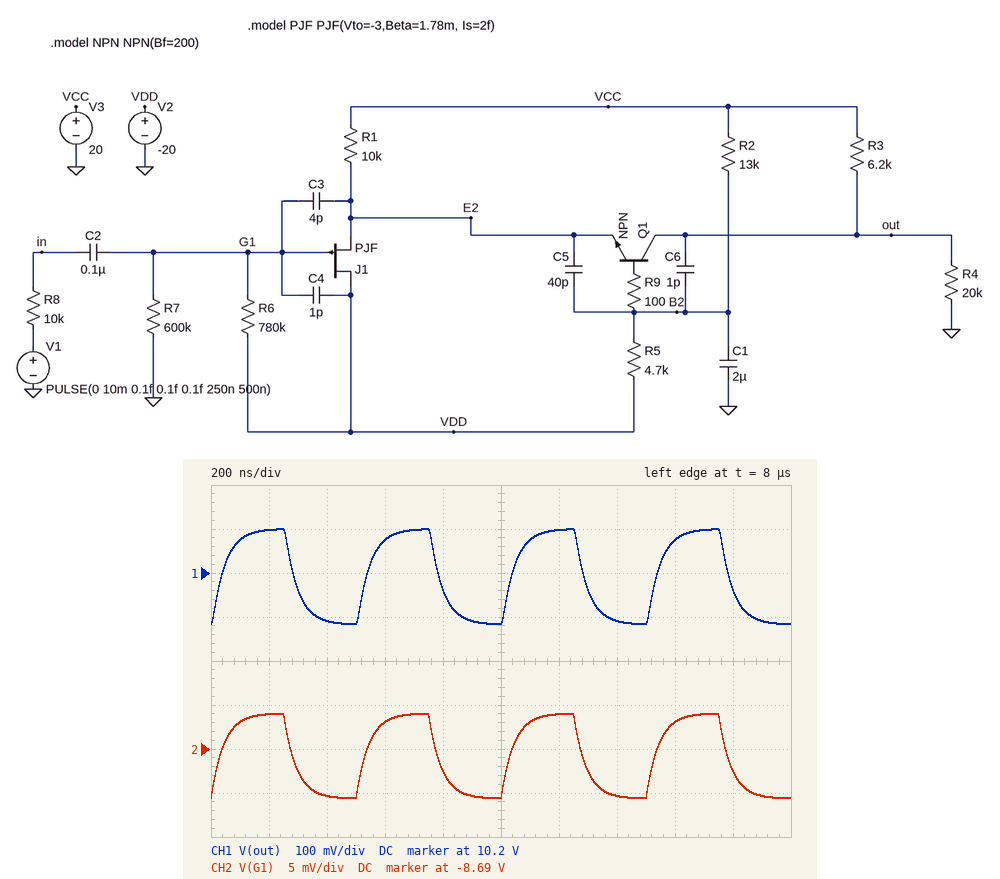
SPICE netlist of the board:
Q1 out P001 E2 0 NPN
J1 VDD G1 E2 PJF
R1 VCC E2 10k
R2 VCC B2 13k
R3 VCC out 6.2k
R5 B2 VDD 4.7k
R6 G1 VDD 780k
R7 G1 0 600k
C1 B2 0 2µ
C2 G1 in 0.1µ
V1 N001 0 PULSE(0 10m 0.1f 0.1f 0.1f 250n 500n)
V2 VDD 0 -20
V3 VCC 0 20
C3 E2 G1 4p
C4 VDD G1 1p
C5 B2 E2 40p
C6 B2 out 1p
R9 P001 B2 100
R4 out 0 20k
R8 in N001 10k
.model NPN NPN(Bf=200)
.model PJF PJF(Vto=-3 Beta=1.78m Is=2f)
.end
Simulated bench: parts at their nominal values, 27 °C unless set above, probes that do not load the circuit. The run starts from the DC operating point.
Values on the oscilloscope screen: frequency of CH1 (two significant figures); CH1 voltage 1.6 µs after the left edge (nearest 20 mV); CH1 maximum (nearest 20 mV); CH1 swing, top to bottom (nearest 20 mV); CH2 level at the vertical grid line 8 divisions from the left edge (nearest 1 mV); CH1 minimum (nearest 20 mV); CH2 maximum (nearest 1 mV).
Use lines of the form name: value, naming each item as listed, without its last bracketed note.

frequency of CH1: 2.0 MHz
CH1 voltage 1.6 µs after the left edge: 10.28 V
CH1 maximum: 10.30 V
CH1 swing, top to bottom: 220 mV
CH2 level at the vertical grid line 8 divisions from the left edge: -8.687 V
CH1 minimum: 10.08 V
CH2 maximum: -8.686 V
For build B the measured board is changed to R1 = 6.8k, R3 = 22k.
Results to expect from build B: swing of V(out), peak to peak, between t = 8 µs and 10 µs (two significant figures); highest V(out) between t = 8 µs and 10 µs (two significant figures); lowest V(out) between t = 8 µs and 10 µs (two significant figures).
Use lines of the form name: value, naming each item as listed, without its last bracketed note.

swing of V(out), peak to peak, between t = 8 µs and 10 µs: 230 mV
highest V(out) between t = 8 µs and 10 µs: 8.6 V
lowest V(out) between t = 8 µs and 10 µs: 8.3 V
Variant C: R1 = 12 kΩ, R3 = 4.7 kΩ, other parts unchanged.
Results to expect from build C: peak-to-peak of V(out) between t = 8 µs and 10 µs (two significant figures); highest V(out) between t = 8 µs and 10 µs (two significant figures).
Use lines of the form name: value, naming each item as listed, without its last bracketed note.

peak-to-peak of V(out) between t = 8 µs and 10 µs: 180 mV
highest V(out) between t = 8 µs and 10 µs: 11 V
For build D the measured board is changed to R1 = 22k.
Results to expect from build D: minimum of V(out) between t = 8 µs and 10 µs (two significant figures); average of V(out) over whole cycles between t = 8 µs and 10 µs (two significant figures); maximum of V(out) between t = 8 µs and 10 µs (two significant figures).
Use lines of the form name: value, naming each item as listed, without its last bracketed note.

minimum of V(out) between t = 8 µs and 10 µs: 3.5 V
average of V(out) over whole cycles between t = 8 µs and 10 µs: 3.6 V
maximum of V(out) between t = 8 µs and 10 µs: 3.7 V
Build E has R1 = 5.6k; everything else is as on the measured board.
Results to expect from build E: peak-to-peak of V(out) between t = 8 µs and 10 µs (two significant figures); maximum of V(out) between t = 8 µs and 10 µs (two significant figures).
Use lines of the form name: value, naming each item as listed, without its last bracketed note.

peak-to-peak of V(out) between t = 8 µs and 10 µs: 1.2 mV
maximum of V(out) between t = 8 µs and 10 µs: 15 V
